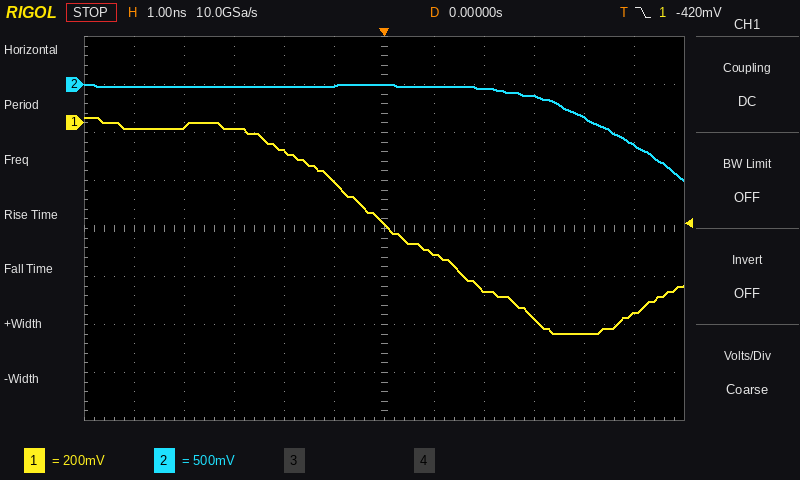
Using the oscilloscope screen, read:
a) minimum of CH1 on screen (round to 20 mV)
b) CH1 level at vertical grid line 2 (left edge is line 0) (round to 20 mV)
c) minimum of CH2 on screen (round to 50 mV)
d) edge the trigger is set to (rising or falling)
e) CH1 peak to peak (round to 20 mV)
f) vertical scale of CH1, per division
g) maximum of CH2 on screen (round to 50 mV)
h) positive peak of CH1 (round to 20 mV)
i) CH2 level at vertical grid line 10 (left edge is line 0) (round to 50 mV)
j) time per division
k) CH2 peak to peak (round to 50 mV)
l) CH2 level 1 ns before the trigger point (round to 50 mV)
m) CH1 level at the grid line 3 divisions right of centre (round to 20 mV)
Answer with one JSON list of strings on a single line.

["-880 mV", "-20 mV", "-1.00 V", "falling", "900 mV", "200 mV", "0 mV", "20 mV", "-350 mV", "1 ns", "1.00 V", "0 mV", "-820 mV"]
